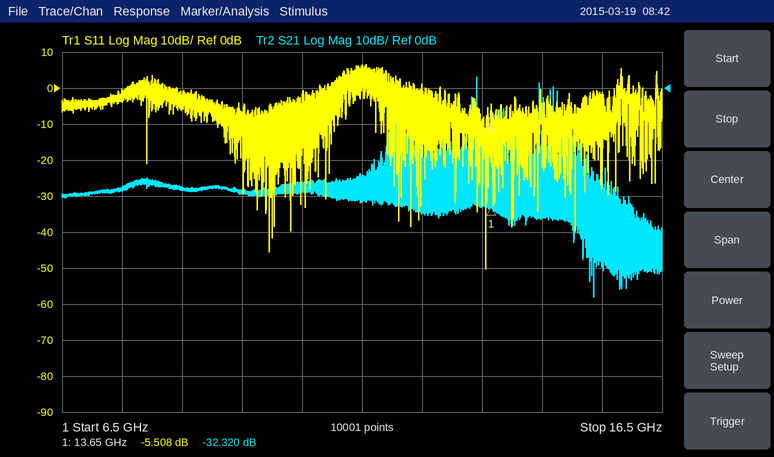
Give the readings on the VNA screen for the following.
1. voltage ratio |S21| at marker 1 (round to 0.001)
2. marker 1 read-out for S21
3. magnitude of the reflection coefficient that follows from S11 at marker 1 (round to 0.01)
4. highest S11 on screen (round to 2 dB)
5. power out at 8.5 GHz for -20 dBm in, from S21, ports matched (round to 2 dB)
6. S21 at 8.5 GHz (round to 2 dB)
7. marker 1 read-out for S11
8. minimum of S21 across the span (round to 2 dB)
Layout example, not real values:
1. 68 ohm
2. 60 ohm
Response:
1. 0.024
2. -32.320 dB
3. 0.53
4. 6 dB
5. -48 dBm
6. -28 dB
7. -5.508 dB
8. -58 dB
